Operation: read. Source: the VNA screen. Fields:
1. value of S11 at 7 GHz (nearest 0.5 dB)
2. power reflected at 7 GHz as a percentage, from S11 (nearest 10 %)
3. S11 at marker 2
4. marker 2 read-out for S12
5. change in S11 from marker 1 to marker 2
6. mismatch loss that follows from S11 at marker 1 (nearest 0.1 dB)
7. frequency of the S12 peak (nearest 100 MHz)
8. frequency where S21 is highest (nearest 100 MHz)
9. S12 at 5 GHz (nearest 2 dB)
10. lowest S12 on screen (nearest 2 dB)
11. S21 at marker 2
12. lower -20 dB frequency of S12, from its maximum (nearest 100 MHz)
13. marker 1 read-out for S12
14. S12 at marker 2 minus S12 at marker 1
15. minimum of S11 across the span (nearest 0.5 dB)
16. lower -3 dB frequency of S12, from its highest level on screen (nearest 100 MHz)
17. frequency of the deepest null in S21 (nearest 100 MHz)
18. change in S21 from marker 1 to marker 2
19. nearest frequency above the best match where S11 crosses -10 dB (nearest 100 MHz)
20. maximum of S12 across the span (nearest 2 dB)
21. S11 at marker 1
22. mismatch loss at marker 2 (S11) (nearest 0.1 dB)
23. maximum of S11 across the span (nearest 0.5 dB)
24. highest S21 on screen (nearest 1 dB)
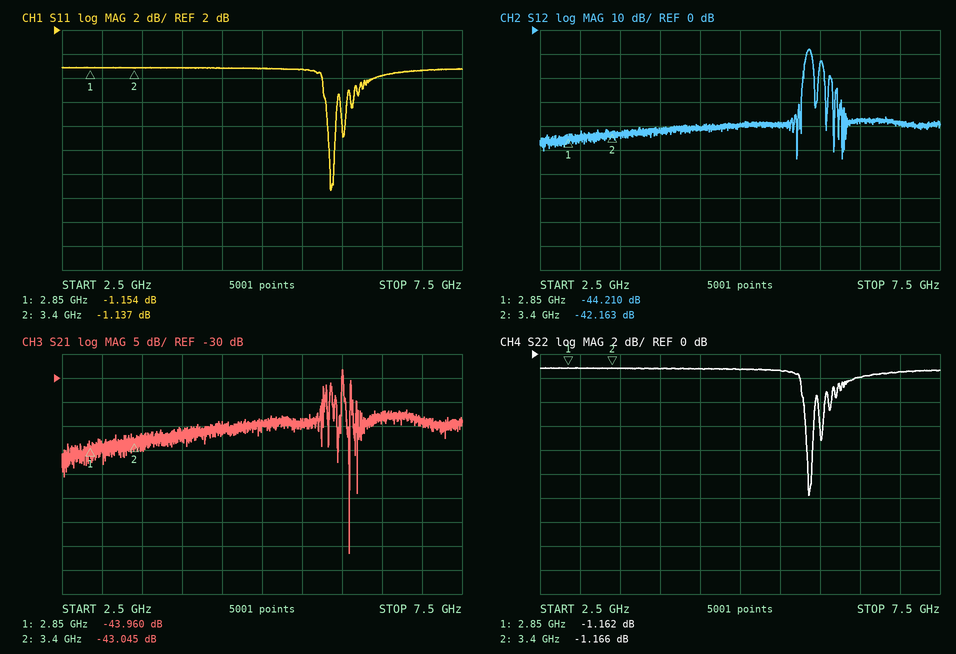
-1.5 dB
70 %
-1.137 dB
-42.163 dB
0.017 dB
6.3 dB
5.9 GHz
6.0 GHz
-40 dB
-54 dB
-43.045 dB
5.8 GHz
-44.210 dB
2.047 dB
-11.5 dB
5.8 GHz
6.1 GHz
0.915 dB
5.9 GHz
-8 dB
-1.154 dB
6.4 dB
-1.0 dB
-28 dB
